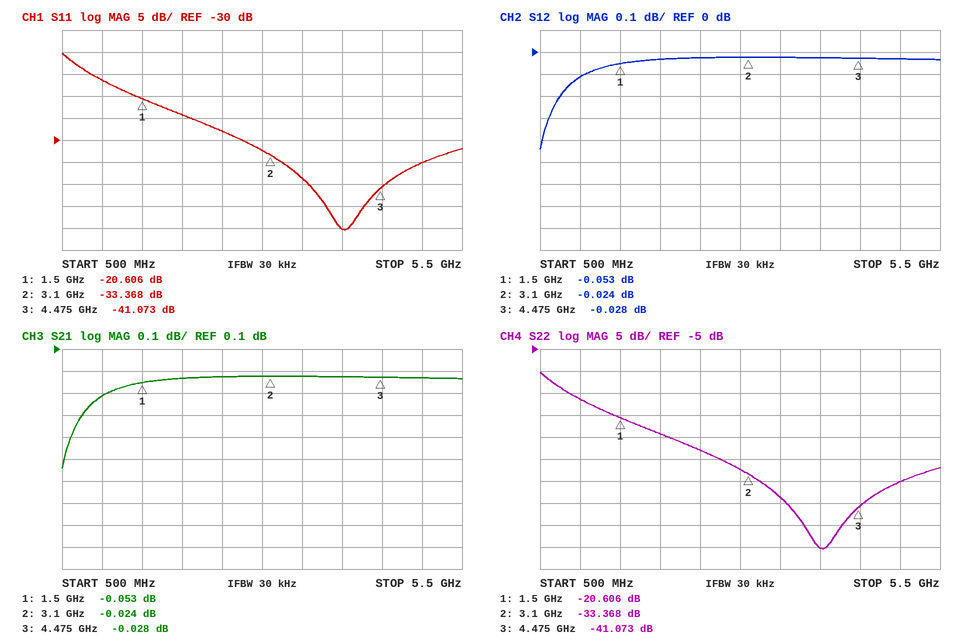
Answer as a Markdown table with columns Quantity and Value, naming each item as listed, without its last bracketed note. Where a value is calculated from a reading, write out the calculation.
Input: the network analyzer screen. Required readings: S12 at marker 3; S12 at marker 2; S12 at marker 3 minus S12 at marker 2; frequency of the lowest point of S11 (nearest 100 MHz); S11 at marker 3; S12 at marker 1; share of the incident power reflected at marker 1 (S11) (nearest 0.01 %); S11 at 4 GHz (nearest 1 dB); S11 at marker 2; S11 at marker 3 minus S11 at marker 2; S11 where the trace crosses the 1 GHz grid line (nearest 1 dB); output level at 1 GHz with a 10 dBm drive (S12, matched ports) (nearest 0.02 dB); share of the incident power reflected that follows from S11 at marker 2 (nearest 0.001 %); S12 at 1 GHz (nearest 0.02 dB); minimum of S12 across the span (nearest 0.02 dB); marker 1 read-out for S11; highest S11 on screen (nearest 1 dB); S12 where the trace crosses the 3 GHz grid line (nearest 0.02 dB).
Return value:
| Quantity | Value |
|---|---|
| S12 at marker 3 | -0.028 dB |
| S12 at marker 2 | -0.024 dB |
| S12 at marker 3 minus S12 at marker 2 | -0.028 − (-0.024) = -0.004 dB |
| frequency of the lowest point of S11 | 4.0 GHz |
| S11 at marker 3 | -41.073 dB |
| S12 at marker 1 | -0.053 dB |
| share of the incident power reflected at marker 1 (S11) | 10^(-20.606/10) ≈ 0.87 % |
| S11 at 4 GHz | -50 dB |
| S11 at marker 2 | -33.368 dB |
| S11 at marker 3 minus S11 at marker 2 | -41.073 − (-33.368) = -7.705 dB |
| S11 where the trace crosses the 1 GHz grid line | -16 dB |
| output level at 1 GHz with a 10 dBm drive (S12, matched ports) | 10 dBm + (-0.12 dB) = 9.88 dBm |
| share of the incident power reflected that follows from S11 at marker 2 | 10^(-33.368/10) ≈ 0.046 % |
| S12 at 1 GHz | -0.12 dB |
| minimum of S12 across the span | -0.44 dB |
| marker 1 read-out for S11 | -20.606 dB |
| highest S11 on screen | -10 dB |
| S12 where the trace crosses the 3 GHz grid line | -0.02 dB |
